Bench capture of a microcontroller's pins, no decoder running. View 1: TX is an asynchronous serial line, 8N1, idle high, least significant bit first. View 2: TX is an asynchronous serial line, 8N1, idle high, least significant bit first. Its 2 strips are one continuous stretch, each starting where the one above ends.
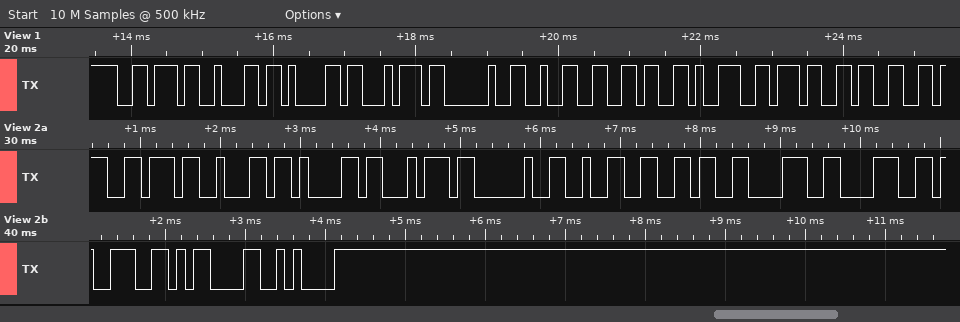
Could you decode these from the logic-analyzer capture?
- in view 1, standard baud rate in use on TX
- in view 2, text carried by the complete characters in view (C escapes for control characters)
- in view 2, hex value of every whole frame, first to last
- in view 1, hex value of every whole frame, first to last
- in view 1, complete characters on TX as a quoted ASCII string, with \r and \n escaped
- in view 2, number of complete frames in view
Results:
9600 baud
"vbat 26889\r\n"
76 62 61 74 20 32 36 38 38 39 0D 0A
0x76 0x62 0x61 0x74 0x20 0x32 0x36 0x39 0x37 0x33
"vbat 26973"
12
